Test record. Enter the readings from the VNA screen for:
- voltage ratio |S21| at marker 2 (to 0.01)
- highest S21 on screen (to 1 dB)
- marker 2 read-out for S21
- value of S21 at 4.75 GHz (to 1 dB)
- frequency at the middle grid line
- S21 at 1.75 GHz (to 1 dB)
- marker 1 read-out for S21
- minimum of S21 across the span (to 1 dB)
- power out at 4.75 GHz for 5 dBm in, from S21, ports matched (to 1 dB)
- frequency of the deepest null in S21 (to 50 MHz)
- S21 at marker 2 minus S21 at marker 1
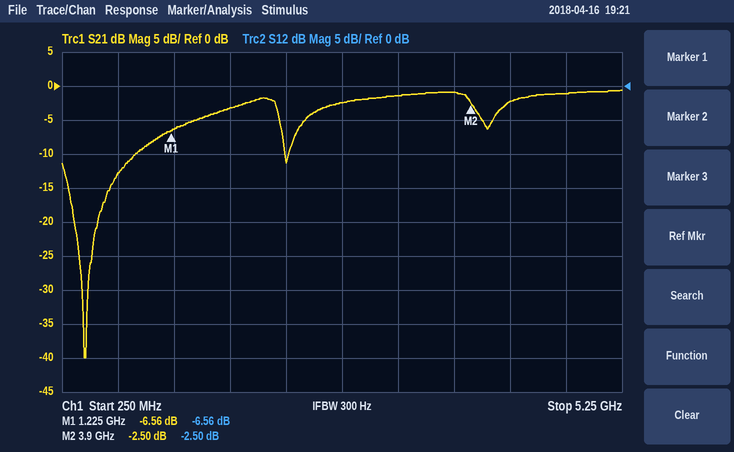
0.75
-1 dB
-2.50 dB
-1 dB
2.75 GHz
-3 dB
-6.56 dB
-40 dB
4 dBm
450 MHz
4.06 dB
